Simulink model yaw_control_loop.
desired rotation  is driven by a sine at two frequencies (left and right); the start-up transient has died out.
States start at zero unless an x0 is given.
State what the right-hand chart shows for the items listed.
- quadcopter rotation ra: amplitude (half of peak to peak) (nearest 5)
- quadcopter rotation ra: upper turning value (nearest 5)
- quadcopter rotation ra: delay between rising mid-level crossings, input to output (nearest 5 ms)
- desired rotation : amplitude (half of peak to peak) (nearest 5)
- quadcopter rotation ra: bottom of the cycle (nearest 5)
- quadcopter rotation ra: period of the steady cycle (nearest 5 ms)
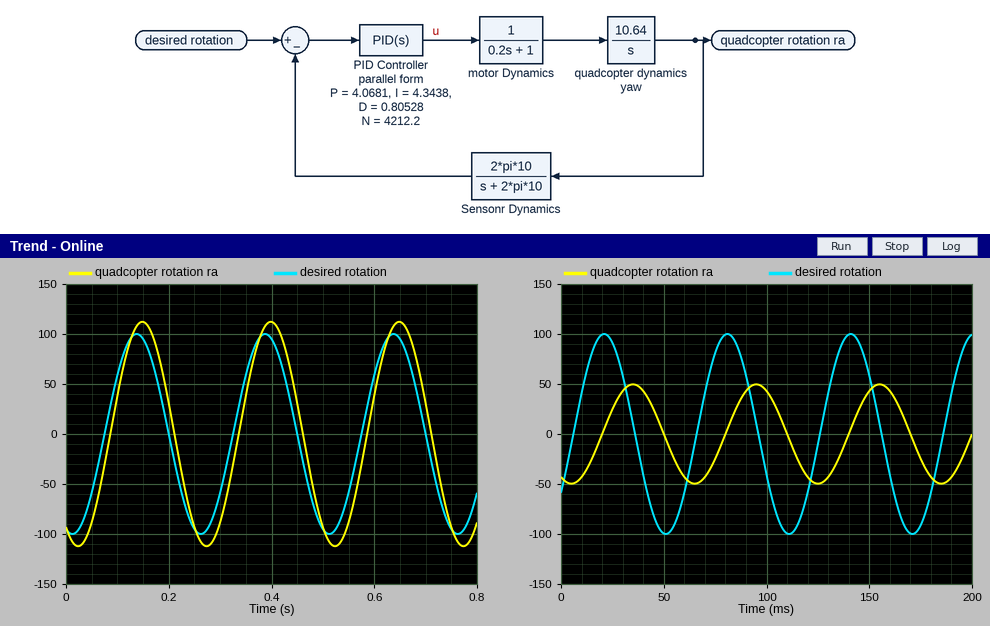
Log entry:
50
50
15 ms
100
-50
60 ms
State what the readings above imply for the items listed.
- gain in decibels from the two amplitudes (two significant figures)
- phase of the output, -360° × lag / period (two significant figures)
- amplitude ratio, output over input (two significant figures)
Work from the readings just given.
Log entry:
-6.0 dB
-90°
0.50
